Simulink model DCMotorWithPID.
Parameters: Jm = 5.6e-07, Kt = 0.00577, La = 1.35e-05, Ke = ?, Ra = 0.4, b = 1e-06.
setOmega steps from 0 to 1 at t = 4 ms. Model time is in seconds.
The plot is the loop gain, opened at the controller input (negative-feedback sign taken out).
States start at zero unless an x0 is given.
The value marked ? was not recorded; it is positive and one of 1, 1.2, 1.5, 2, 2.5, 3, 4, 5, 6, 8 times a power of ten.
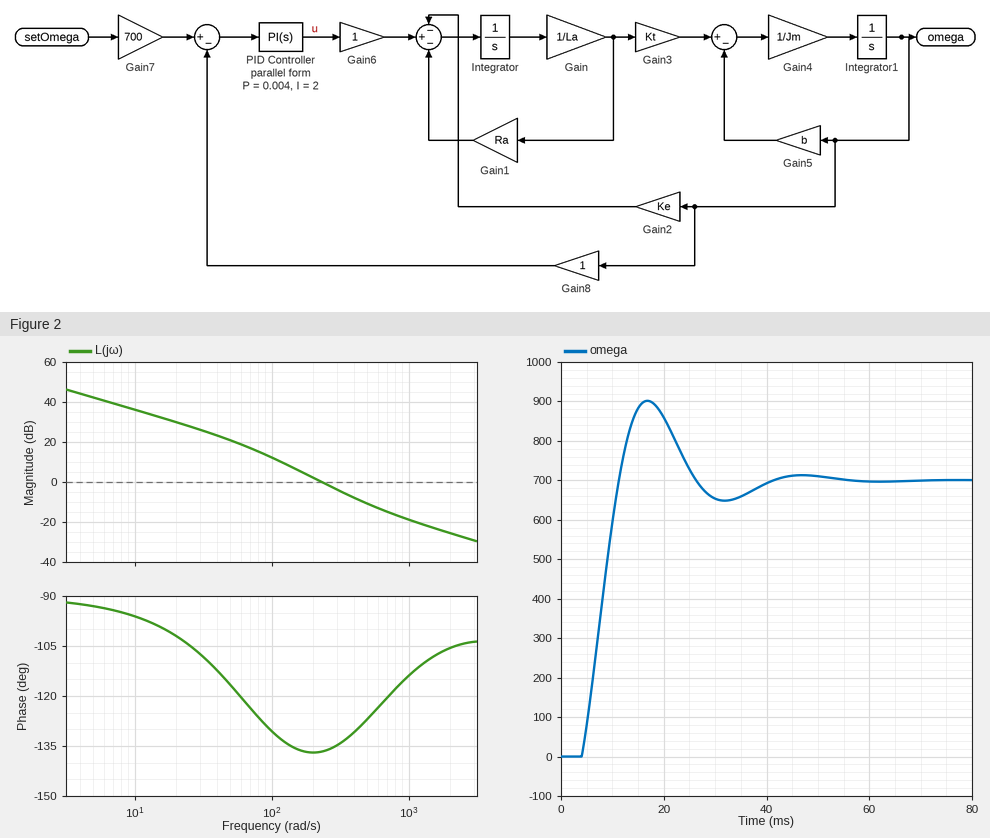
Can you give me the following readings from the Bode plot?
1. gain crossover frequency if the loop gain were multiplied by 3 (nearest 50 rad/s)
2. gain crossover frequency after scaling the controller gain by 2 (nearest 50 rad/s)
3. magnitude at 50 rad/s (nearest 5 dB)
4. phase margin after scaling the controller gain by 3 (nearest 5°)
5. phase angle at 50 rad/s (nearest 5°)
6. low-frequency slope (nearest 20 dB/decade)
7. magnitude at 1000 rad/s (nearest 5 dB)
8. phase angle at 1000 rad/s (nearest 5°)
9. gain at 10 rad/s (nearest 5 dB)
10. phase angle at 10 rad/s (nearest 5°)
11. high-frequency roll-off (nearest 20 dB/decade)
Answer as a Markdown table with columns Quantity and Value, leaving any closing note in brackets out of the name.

| Quantity | Value |
|---|---|
| gain crossover frequency if the loop gain were multiplied by 3 | 450 rad/s |
| gain crossover frequency after scaling the controller gain by 2 | 350 rad/s |
| magnitude at 50 rad/s | 20 dB |
| phase margin after scaling the controller gain by 3 | 50° |
| phase angle at 50 rad/s | -115° |
| low-frequency slope | -20 dB/decade |
| magnitude at 1000 rad/s | -20 dB |
| phase angle at 1000 rad/s | -115° |
| gain at 10 rad/s | 35 dB |
| phase angle at 10 rad/s | -95° |
| high-frequency roll-off | -20 dB/decade |
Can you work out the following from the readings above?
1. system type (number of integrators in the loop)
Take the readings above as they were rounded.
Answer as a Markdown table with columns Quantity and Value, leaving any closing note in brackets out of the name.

| Quantity | Value |
|---|---|
| system type | 1 |
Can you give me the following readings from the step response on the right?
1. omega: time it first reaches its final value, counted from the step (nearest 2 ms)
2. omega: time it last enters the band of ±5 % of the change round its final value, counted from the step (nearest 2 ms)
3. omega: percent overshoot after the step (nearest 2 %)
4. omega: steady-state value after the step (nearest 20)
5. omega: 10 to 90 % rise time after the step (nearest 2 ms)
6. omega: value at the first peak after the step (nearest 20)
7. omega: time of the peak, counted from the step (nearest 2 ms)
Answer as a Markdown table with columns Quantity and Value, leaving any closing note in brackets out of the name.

| Quantity | Value |
|---|---|
| omega: time it first reaches its final value, counted from the step | 8 ms |
| omega: time it last enters the band of ±5 % of the change round its final value, counted from the step | 32 ms |
| omega: percent overshoot after the step | 28 % |
| omega: steady-state value after the step | 700 |
| omega: 10 to 90 % rise time after the step | 6 ms |
| omega: value at the first peak after the step | 900 |
| omega: time of the peak, counted from the step | 12 ms |
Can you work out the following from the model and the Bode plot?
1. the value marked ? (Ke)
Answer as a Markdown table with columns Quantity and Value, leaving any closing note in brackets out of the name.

| Quantity | Value |
|---|---|
| the value marked ? | 0.003 |
